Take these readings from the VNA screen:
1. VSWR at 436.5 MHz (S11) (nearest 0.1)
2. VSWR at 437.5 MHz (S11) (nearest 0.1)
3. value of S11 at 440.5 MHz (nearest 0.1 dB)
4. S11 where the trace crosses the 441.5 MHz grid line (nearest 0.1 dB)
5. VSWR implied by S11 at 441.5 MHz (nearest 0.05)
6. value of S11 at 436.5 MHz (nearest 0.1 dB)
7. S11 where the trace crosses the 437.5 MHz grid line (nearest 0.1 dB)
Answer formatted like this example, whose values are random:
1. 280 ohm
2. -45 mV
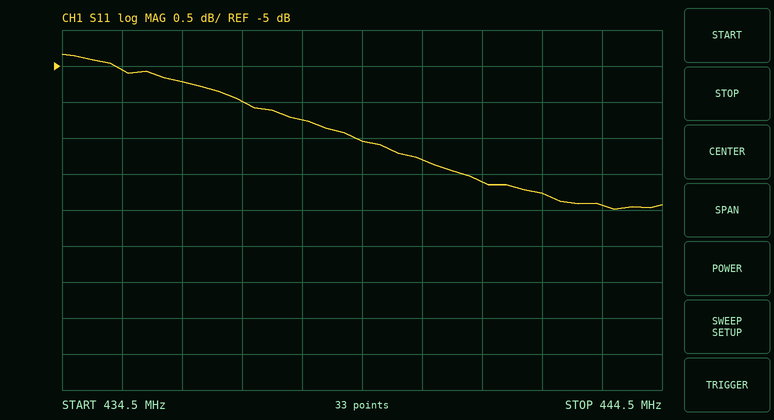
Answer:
1. 3.4
2. 3.3
3. -6.3 dB
4. -6.6 dB
5. 2.75
6. -5.2 dB
7. -5.5 dB
